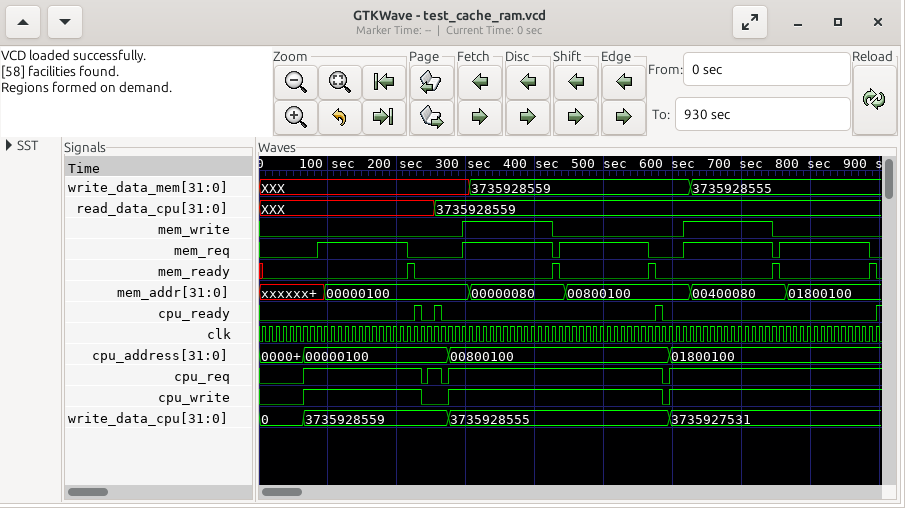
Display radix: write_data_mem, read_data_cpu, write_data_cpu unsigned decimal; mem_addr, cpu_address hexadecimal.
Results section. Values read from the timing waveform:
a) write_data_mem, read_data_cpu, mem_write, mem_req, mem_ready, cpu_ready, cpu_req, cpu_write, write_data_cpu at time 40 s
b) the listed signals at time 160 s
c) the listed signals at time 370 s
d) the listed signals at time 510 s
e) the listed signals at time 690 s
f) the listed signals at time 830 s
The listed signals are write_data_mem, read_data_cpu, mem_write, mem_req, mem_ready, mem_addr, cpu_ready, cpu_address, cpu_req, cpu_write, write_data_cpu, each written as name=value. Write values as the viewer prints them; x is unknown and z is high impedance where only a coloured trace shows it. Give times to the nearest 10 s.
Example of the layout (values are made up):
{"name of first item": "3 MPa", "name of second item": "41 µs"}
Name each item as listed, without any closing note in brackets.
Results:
{"write_data_mem, read_data_cpu, mem_write, mem_req, mem_ready, cpu_ready, cpu_req, cpu_write, write_data_cpu at time 40 s": "write_data_mem=XXX, read_data_cpu=XXX, mem_write=0, mem_req=0, mem_ready=0, cpu_ready=0, cpu_req=0, cpu_write=0, write_data_cpu=0", "the listed signals at time 160 s": "write_data_mem=XXX, read_data_cpu=XXX, mem_write=0, mem_req=1, mem_ready=0, mem_addr=00000100, cpu_ready=0, cpu_address=00000100, cpu_req=1, cpu_write=1, write_data_cpu=3735928559", "the listed signals at time 370 s": "write_data_mem=3735928559, read_data_cpu=3735928559, mem_write=1, mem_req=1, mem_ready=0, mem_addr=00000080, cpu_ready=0, cpu_address=00800100, cpu_req=1, cpu_write=1, write_data_cpu=3735928555", "the listed signals at time 510 s": "write_data_mem=3735928559, read_data_cpu=3735928559, mem_write=0, mem_req=1, mem_ready=0, mem_addr=00800100, cpu_ready=0, cpu_address=00800100, cpu_req=1, cpu_write=1, write_data_cpu=3735928555", "the listed signals at time 690 s": "write_data_mem=3735928555, read_data_cpu=3735928559, mem_write=1, mem_req=1, mem_ready=0, mem_addr=00400080, cpu_ready=0, cpu_address=01800100, cpu_req=1, cpu_write=1, write_data_cpu=3735927531", "the listed signals at time 830 s": "write_data_mem=3735928555, read_data_cpu=3735928559, mem_write=0, mem_req=1, mem_ready=0, mem_addr=01800100, cpu_ready=0, cpu_address=01800100, cpu_req=1, cpu_write=1, write_data_cpu=3735927531"}
